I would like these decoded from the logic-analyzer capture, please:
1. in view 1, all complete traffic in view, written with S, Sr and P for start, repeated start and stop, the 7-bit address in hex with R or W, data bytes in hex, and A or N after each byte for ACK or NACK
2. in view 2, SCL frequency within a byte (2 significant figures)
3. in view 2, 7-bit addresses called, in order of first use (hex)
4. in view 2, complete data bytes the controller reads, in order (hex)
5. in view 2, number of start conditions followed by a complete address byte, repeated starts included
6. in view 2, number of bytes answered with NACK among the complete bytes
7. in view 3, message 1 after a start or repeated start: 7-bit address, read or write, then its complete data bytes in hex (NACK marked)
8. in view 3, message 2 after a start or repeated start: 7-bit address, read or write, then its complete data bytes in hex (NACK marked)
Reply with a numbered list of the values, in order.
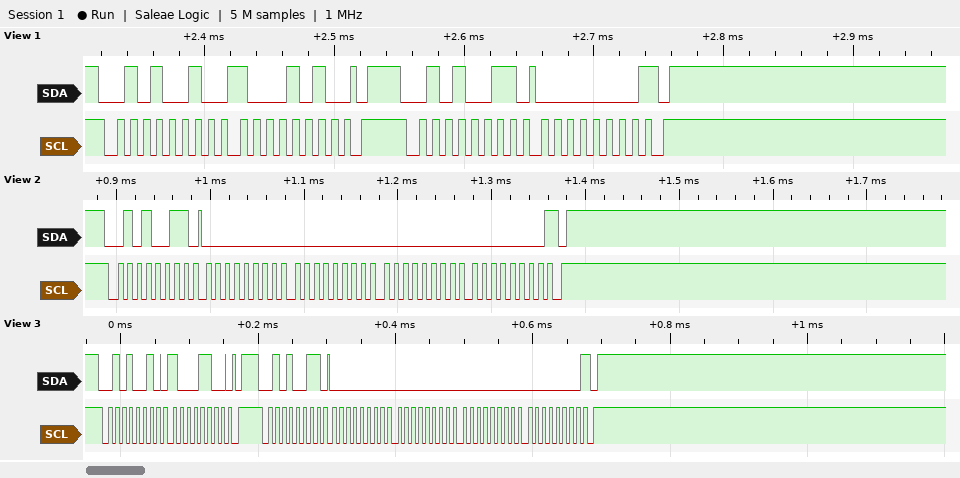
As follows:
1. S 29W A 8A A P S 29R A 00 N P
2. 100 kHz
3. 0x29
4. 00 00 00 00
5. 1
6. 1
7. 0x29 write: 8C
8. 0x29 read: 00 00 00 00 NACK
